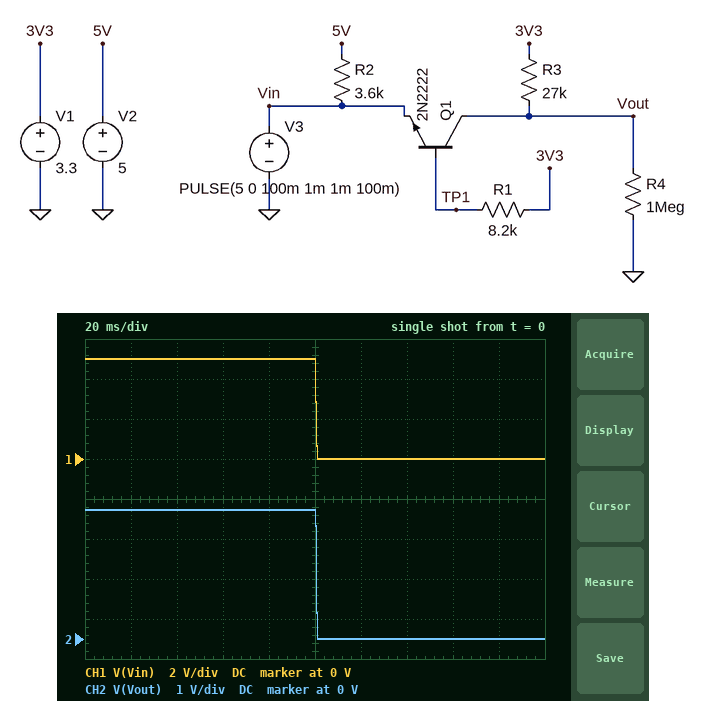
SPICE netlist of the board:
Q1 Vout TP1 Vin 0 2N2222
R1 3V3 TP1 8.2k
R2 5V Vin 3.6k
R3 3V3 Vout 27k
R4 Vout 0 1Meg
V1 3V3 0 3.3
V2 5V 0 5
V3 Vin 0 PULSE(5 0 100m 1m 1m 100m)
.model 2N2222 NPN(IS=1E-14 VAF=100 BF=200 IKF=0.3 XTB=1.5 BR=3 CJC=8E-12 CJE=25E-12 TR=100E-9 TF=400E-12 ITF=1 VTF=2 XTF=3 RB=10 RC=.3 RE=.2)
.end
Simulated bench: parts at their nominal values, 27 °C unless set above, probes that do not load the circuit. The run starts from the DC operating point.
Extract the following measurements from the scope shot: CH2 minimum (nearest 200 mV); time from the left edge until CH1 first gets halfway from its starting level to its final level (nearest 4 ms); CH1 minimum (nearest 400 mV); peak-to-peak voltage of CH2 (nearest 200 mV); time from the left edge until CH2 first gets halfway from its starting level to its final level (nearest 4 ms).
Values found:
0 V
100 ms
0 V
3.2 V
100 ms
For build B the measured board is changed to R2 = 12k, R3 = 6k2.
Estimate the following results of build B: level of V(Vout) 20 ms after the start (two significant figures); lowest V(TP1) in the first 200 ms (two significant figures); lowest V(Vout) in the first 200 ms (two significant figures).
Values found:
3.3 V
670 mV
17 mV
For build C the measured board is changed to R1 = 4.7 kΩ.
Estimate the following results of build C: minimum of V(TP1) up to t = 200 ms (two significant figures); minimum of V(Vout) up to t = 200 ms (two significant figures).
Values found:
680 mV
9.1 mV
